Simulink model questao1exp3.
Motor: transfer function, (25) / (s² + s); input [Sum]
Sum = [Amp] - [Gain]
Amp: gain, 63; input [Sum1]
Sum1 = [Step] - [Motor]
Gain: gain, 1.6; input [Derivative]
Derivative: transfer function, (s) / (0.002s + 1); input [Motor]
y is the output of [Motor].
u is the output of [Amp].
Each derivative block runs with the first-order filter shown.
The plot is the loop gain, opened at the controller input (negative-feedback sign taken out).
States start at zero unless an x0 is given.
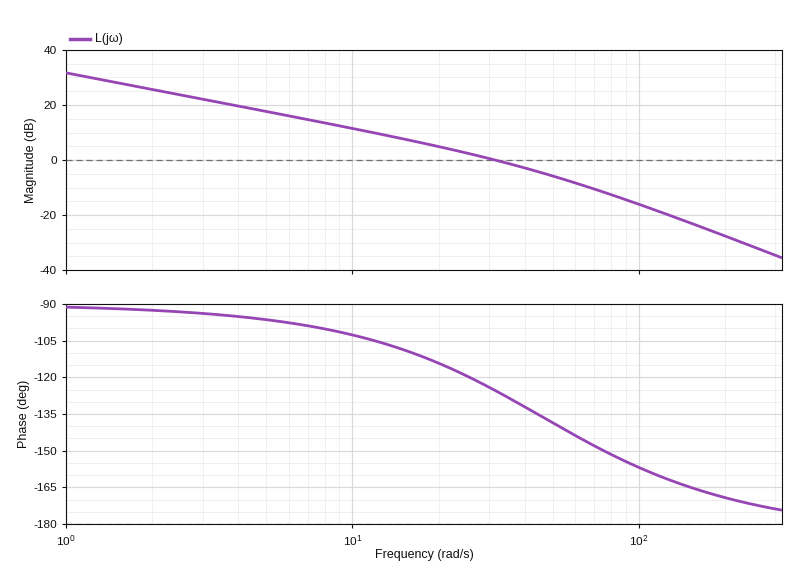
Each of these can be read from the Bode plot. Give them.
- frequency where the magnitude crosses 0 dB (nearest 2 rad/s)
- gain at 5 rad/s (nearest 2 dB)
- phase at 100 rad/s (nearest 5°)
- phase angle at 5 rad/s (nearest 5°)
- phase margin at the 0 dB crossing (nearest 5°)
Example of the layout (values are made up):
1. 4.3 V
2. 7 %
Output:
1. 32 rad/s
2. 18 dB
3. -155°
4. -95°
5. 55°
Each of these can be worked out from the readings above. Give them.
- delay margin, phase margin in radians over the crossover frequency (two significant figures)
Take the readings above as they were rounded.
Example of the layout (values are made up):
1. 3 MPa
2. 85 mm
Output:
1. 0.030 s
